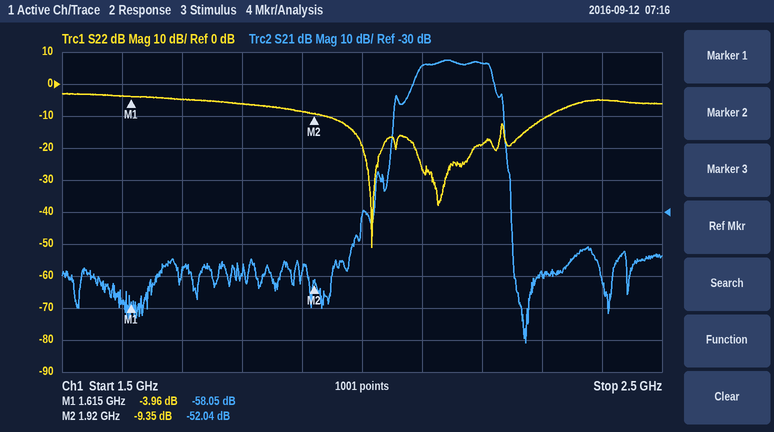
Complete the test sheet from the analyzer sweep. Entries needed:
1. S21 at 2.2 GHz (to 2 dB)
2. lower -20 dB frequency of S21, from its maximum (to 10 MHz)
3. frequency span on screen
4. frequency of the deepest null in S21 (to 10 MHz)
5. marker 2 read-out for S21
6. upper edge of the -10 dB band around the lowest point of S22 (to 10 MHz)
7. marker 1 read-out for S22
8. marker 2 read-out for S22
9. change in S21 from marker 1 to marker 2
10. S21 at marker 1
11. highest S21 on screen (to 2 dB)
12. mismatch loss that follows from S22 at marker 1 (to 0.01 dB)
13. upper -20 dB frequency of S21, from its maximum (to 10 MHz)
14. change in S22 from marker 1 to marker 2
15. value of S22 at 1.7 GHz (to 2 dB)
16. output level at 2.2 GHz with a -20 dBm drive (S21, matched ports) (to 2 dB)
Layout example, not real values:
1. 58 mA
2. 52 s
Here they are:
1. 16 dB
2. 2.05 GHz
3. 1 GHz
4. 2.27 GHz
5. -52.04 dB
6. 2.31 GHz
7. -3.96 dB
8. -9.35 dB
9. 6.01 dB
10. -58.05 dB
11. 18 dB
12. 2.23 dB
13. 2.24 GHz
14. -5.39 dB
15. -4 dB
16. -4 dBm
